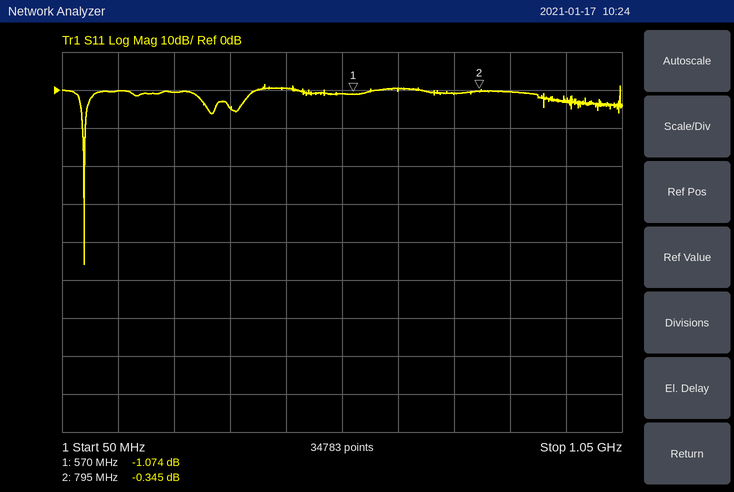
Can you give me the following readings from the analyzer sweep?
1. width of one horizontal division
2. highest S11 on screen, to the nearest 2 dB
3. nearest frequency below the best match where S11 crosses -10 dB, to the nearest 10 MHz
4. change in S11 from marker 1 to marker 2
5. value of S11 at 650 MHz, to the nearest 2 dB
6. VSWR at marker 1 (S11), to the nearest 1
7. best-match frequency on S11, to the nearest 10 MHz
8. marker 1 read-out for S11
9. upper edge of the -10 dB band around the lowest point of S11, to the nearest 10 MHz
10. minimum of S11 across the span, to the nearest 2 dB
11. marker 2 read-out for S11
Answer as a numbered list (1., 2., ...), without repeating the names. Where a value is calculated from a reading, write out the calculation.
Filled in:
1. 100 MHz
2. 2 dB
3. 90 MHz
4. -0.345 − (-1.074) = 0.729 dB
5. 0 dB
6. (1 + 0.8837)/(1 − 0.8837) ≈ 16
7. 90 MHz
8. -1.074 dB
9. 90 MHz
10. -46 dB
11. -0.345 dB
